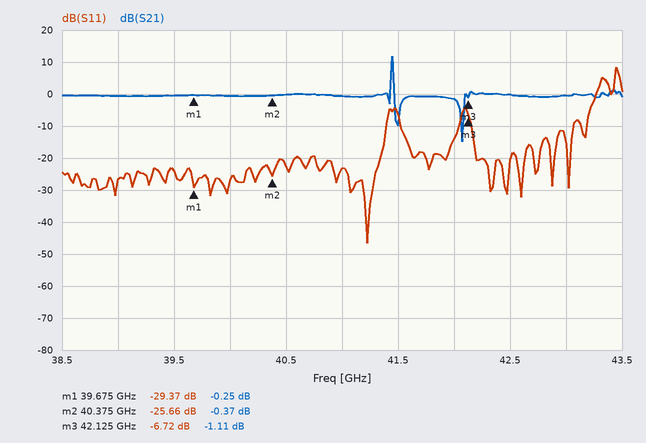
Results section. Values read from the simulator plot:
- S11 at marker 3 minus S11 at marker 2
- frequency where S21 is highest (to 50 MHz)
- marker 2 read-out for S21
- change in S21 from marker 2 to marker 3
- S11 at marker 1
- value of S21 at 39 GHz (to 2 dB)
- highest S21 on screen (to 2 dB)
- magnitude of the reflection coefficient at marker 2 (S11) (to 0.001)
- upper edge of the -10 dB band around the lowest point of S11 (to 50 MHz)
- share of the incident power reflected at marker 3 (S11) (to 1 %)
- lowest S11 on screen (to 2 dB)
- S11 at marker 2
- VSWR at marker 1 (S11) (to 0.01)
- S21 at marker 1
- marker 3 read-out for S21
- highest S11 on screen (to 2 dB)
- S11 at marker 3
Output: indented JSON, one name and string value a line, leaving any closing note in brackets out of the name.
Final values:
{
  "S11 at marker 3 minus S11 at marker 2": "18.94 dB",
  "frequency where S21 is highest": "41.45 GHz",
  "marker 2 read-out for S21": "-0.37 dB",
  "change in S21 from marker 2 to marker 3": "-0.74 dB",
  "S11 at marker 1": "-29.37 dB",
  "value of S21 at 39 GHz": "0 dB",
  "highest S21 on screen": "12 dB",
  "magnitude of the reflection coefficient at marker 2 (S11)": "0.052",
  "upper edge of the -10 dB band around the lowest point of S11": "41.40 GHz",
  "share of the incident power reflected at marker 3 (S11)": "21 %",
  "lowest S11 on screen": "-46 dB",
  "S11 at marker 2": "-25.66 dB",
  "VSWR at marker 1 (S11)": "1.07",
  "S21 at marker 1": "-0.25 dB",
  "marker 3 read-out for S21": "-1.11 dB",
  "highest S11 on screen": "8 dB",
  "S11 at marker 3": "-6.72 dB"
}
